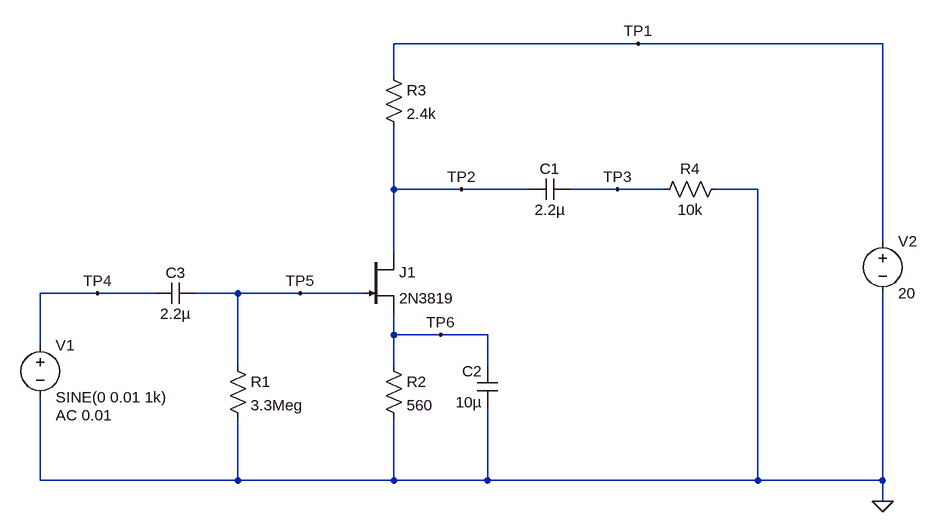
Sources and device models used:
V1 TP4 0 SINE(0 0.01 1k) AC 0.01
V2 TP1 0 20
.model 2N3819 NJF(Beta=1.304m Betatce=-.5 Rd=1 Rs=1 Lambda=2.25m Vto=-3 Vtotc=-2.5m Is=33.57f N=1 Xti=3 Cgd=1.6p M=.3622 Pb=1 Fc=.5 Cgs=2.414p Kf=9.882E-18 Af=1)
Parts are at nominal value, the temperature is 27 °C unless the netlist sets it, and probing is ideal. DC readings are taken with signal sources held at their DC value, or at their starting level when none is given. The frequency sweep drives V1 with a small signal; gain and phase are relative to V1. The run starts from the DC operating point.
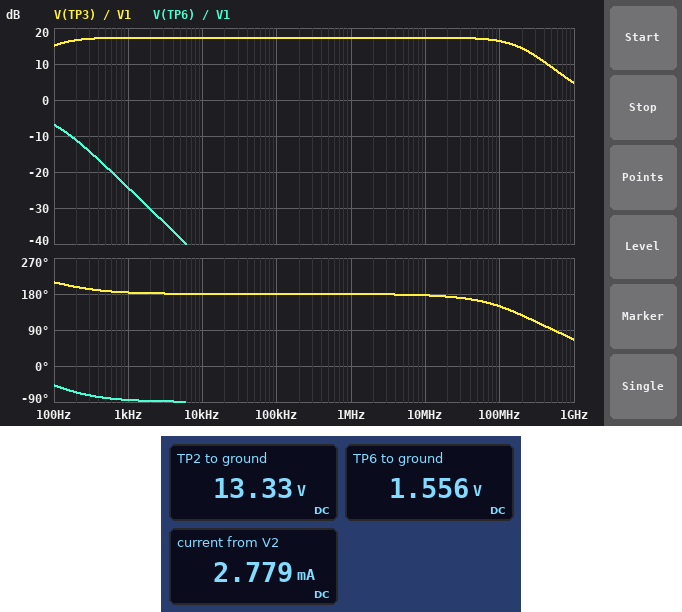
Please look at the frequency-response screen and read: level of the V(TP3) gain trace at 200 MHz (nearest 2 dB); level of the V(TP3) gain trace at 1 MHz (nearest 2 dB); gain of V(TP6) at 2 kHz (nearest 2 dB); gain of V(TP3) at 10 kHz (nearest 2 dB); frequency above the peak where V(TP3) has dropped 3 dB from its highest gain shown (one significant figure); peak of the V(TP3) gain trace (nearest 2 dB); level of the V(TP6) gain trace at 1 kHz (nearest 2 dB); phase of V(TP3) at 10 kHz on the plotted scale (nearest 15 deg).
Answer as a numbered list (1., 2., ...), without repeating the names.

1. 14 dB
2. 18 dB
3. -30 dB
4. 18 dB
5. 200 MHz
6. 18 dB
7. -24 dB
8. 180 deg
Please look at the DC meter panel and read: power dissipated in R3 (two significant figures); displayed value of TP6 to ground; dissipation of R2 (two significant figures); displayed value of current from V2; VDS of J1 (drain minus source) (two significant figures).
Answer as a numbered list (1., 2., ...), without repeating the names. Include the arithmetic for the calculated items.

1. (20 V - 13.33 V)^2 / 2.4 kΩ = 19 mW
2. 1.556 V
3. (1.556 V)^2 / 560 Ω = 4.3 mW
4. 2.779 mA
5. 13.33 V - 1.556 V = 12 V
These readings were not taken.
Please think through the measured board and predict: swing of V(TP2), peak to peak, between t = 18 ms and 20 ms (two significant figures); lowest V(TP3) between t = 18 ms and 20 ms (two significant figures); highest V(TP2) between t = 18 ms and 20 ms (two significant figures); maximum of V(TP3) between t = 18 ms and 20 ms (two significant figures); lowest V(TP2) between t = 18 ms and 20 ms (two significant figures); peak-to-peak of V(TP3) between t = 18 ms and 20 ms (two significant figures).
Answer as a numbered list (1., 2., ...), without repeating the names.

1. 150 mV
2. -73 mV
3. 13 V
4. 73 mV
5. 13 V
6. 150 mV
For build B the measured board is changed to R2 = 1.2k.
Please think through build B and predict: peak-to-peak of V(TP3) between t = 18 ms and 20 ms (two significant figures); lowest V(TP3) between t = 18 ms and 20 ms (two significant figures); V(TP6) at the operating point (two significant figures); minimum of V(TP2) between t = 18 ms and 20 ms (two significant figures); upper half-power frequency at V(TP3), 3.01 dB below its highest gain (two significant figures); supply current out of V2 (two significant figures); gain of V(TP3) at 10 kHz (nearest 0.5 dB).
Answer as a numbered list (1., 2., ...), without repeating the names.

1. 110 mV
2. -56 mV
3. 1.9 V
4. 16 V
5. 220 MHz
6. 1.6 mA
7. 15.0 dB
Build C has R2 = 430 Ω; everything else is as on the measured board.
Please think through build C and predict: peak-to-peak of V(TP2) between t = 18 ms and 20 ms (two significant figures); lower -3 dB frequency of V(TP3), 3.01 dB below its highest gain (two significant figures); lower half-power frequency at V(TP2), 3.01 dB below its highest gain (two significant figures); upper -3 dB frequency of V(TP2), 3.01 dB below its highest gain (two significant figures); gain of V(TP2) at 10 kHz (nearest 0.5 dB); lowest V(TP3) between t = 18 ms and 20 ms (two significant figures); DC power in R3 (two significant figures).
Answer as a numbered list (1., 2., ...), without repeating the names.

1. 160 mV
2. 89 Hz
3. 88 Hz
4. 190 MHz
5. 18.0 dB
6. -80 mV
7. 26 mW
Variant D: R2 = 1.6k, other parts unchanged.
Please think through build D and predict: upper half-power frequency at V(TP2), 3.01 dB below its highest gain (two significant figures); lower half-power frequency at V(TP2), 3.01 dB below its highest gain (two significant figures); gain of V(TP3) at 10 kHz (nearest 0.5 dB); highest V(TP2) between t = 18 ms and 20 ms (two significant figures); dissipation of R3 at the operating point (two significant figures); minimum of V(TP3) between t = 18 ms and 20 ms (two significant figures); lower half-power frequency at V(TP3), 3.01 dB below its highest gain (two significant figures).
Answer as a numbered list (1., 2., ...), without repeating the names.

1. 230 MHz
2. 49 Hz
3. 14.0 dB
4. 17 V
5. 3.9 mW
6. -50 mV
7. 50 Hz
